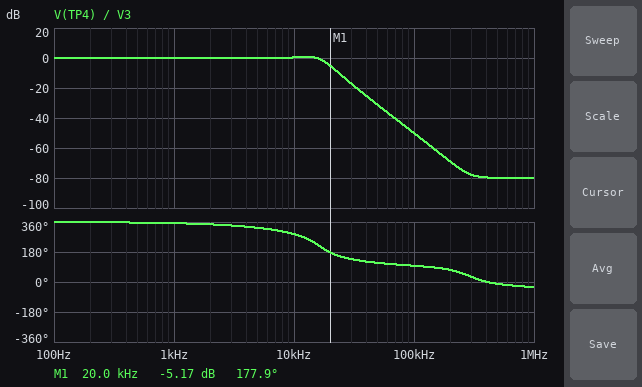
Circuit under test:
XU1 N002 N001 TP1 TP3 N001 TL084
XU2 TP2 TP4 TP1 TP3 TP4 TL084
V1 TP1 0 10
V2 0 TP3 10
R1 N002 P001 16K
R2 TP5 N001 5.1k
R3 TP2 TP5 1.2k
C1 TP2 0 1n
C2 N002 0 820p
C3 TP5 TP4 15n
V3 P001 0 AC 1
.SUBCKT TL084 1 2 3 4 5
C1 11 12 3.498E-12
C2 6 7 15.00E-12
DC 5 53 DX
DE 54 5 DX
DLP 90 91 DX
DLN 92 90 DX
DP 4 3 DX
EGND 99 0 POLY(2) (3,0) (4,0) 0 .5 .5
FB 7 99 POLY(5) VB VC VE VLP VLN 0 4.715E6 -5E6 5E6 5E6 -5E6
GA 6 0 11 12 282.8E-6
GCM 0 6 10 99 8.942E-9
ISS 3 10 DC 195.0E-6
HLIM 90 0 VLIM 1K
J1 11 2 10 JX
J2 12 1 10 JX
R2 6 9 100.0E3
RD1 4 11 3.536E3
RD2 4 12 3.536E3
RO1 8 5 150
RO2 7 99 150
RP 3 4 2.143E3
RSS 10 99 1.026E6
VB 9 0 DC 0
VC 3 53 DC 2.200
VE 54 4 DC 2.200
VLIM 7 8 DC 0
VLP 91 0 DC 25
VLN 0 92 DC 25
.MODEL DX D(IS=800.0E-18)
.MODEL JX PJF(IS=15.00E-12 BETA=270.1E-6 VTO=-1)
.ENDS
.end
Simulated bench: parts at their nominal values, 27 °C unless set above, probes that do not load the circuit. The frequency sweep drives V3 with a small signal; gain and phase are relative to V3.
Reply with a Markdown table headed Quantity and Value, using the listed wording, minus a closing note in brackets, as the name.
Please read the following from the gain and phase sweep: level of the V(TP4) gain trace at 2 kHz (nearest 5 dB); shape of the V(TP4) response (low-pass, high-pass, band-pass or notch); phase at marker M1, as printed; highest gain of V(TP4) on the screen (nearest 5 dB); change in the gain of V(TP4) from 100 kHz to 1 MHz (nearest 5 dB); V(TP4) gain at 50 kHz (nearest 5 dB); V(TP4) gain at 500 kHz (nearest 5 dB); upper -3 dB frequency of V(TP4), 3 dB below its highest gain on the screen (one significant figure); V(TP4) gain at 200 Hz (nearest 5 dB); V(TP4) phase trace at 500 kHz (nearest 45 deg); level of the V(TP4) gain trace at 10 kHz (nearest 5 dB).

| Quantity | Value |
|---|---|
| level of the V(TP4) gain trace at 2 kHz | 0 dB |
| shape of the V(TP4) response | low-pass |
| phase at marker M1, as printed | 177.9 deg |
| highest gain of V(TP4) on the screen | 0 dB |
| change in the gain of V(TP4) from 100 kHz to 1 MHz | -30 dB |
| V(TP4) gain at 50 kHz | -30 dB |
| V(TP4) gain at 500 kHz | -80 dB |
| upper -3 dB frequency of V(TP4), 3 dB below its highest gain on the screen | 20 kHz |
| V(TP4) gain at 200 Hz | 0 dB |
| V(TP4) phase trace at 500 kHz | 0 deg |
| level of the V(TP4) gain trace at 10 kHz | 0 dB |
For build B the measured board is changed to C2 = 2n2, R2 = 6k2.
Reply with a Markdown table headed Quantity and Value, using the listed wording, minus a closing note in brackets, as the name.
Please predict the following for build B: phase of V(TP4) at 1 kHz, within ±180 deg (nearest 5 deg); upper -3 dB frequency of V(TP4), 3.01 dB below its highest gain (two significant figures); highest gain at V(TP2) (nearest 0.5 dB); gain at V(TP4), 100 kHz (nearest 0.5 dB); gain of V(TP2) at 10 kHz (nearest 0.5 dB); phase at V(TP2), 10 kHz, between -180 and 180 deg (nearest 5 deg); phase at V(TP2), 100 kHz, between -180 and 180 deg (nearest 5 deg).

| Quantity | Value |
|---|---|
| phase of V(TP4) at 1 kHz, within ±180 deg | -15 deg |
| upper -3 dB frequency of V(TP4), 3.01 dB below its highest gain | 5.5 kHz |
| highest gain at V(TP2) | 0 dB |
| gain at V(TP4), 100 kHz | -60.5 dB |
| gain of V(TP2) at 10 kHz | -5.0 dB |
| phase at V(TP2), 10 kHz, between -180 and 180 deg | -105 deg |
| phase at V(TP2), 100 kHz, between -180 and 180 deg | 95 deg |
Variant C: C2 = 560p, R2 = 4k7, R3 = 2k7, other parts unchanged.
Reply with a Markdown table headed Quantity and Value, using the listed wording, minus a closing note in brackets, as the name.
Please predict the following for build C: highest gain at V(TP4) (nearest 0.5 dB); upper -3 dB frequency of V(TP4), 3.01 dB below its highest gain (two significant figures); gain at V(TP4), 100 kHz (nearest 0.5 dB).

| Quantity | Value |
|---|---|
| highest gain at V(TP4) | 4.5 dB |
| upper -3 dB frequency of V(TP4), 3.01 dB below its highest gain | 13 kHz |
| gain at V(TP4), 100 kHz | -53.0 dB |
